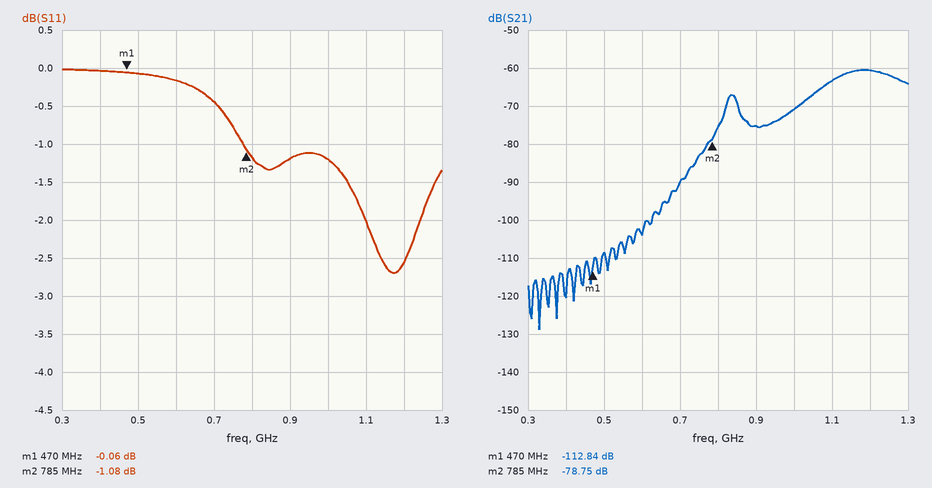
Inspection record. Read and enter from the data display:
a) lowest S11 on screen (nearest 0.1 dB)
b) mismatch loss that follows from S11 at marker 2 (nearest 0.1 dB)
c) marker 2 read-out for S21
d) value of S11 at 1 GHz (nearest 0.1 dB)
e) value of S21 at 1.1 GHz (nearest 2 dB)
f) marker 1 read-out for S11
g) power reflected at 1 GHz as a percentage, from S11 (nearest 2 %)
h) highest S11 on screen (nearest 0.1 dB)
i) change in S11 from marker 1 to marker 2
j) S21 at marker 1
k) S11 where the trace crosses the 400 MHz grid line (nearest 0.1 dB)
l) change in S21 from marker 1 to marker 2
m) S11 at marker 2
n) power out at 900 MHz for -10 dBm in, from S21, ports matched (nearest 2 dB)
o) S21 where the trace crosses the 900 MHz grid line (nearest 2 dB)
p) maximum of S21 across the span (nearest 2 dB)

-2.7 dB
6.6 dB
-78.75 dB
-1.2 dB
-64 dB
-0.06 dB
76 %
0.0 dB
-1.02 dB
-112.84 dB
0.0 dB
34.09 dB
-1.08 dB
-86 dBm
-76 dB
-60 dB
